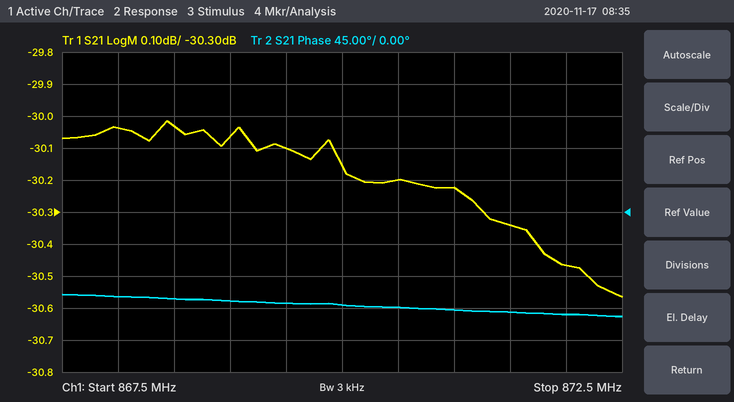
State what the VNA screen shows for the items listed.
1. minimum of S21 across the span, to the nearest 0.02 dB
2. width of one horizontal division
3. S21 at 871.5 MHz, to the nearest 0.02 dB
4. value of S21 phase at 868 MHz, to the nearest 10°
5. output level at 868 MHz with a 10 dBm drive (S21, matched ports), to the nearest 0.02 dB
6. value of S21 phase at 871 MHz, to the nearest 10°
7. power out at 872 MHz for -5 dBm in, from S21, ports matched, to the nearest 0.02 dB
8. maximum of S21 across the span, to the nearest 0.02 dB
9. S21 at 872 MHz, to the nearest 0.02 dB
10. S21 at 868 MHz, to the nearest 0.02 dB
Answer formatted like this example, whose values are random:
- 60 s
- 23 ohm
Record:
- -30.56 dB
- 500 kHz
- -30.34 dB
- -120°
- -20.04 dBm
- -140°
- -35.46 dBm
- -30.02 dB
- -30.46 dB
- -30.04 dB
